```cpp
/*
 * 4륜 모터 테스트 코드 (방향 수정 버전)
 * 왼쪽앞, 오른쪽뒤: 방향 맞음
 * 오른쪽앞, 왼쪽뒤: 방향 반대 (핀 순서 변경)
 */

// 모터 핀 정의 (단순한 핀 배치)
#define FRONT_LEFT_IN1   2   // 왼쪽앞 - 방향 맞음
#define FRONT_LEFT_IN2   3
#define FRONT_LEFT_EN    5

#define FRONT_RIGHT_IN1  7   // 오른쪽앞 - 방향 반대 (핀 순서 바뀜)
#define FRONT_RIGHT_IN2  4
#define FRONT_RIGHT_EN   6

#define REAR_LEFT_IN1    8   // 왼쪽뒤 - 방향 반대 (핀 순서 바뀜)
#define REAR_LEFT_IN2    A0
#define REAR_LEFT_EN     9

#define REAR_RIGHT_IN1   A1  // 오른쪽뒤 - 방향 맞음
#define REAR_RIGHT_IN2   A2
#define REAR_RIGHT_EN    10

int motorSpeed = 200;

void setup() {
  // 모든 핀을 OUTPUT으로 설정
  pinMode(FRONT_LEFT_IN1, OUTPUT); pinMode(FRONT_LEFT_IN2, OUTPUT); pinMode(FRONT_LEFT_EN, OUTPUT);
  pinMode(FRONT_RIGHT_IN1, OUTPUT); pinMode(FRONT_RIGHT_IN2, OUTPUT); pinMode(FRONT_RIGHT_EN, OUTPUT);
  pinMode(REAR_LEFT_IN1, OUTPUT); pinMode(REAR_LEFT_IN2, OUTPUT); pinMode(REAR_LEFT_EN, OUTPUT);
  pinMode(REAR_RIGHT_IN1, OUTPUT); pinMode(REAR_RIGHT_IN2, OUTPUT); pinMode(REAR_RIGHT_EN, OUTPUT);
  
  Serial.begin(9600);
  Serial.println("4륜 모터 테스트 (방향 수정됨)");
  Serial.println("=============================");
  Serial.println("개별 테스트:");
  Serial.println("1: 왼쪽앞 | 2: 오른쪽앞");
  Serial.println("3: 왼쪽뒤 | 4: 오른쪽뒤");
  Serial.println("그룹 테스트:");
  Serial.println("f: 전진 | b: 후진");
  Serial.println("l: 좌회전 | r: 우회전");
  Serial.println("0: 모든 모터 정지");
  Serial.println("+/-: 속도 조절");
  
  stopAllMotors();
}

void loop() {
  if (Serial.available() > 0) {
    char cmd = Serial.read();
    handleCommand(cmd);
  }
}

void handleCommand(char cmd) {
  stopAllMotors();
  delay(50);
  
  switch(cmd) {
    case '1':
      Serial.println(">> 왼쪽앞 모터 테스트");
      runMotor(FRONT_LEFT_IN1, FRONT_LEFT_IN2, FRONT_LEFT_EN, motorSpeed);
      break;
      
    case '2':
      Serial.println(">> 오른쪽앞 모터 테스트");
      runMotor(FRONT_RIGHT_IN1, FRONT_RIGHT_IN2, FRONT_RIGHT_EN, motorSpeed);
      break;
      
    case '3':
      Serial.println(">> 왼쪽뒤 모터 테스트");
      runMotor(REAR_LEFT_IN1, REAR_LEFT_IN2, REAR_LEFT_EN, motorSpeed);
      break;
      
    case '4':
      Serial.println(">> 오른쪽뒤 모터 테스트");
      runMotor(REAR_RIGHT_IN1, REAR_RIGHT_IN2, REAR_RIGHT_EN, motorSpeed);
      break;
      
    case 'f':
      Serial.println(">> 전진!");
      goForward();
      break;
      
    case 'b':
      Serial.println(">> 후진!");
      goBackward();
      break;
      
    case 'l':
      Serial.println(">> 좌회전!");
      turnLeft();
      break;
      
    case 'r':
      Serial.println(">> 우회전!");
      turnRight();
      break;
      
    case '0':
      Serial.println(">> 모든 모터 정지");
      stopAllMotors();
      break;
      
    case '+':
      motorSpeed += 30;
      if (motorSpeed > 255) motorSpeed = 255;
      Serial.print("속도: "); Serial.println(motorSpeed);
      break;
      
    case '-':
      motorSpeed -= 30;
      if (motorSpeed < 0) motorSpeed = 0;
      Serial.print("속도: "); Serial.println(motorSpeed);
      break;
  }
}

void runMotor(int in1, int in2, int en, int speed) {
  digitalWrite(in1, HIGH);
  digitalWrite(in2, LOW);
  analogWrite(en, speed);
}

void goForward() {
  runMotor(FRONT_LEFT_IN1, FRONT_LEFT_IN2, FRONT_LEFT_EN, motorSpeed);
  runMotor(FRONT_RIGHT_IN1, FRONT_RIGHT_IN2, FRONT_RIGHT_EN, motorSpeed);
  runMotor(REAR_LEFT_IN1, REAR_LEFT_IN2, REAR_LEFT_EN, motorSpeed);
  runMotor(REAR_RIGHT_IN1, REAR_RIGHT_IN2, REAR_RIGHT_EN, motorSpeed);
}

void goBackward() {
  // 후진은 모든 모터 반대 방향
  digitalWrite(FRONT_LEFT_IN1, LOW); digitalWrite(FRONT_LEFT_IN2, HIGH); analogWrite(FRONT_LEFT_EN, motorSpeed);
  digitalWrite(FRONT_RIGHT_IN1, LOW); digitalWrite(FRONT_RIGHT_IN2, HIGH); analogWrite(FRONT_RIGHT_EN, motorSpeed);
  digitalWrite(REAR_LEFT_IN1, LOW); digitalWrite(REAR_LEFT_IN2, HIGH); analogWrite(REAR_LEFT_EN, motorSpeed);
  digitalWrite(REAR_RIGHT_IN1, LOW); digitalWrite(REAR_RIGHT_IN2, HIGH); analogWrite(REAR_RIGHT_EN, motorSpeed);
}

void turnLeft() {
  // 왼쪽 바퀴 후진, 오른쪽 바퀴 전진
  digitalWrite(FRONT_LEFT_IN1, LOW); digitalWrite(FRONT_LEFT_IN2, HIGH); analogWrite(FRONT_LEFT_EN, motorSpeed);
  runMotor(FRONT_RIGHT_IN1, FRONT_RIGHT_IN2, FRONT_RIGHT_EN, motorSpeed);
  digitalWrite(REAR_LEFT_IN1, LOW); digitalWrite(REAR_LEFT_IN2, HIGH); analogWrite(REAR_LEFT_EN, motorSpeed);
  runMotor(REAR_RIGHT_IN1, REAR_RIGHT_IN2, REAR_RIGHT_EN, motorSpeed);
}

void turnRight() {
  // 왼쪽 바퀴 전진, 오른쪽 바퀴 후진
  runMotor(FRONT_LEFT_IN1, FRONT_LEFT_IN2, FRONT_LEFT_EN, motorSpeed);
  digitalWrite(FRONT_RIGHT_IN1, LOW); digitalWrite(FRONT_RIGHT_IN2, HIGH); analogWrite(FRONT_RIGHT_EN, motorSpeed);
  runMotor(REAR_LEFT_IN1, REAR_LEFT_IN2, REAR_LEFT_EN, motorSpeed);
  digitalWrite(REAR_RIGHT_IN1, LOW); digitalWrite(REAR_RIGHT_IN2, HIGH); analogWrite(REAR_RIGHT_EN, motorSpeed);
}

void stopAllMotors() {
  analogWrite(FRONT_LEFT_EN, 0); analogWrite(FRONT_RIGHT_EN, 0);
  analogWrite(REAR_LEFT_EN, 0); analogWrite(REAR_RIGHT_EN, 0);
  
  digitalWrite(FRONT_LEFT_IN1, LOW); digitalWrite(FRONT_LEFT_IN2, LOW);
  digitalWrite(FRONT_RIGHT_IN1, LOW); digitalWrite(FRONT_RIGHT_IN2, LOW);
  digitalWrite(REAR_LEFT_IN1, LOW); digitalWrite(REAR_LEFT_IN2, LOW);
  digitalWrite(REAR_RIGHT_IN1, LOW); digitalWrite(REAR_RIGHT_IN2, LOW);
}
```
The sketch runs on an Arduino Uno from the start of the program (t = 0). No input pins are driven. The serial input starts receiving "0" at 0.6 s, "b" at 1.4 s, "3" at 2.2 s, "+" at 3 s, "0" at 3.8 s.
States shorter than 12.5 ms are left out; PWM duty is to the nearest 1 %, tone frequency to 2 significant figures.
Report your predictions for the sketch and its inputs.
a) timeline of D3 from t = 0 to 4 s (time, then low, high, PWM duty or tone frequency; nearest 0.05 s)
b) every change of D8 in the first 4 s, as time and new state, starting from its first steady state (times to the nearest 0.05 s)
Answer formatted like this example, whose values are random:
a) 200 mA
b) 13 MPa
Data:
a) 0 s low; 1.45 s high; 2.2 s low
b) 0 s low; 2.25 s high; 3 s low
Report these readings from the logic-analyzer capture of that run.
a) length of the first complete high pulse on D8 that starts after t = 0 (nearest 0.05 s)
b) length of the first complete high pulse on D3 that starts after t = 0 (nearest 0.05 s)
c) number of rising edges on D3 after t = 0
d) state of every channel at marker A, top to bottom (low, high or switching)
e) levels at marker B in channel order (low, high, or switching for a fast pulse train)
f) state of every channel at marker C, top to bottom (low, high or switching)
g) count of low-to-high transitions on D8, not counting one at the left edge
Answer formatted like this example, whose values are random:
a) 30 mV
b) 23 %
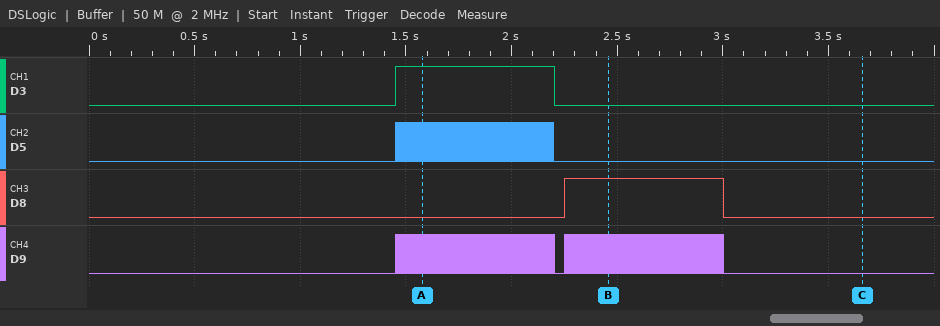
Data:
a) 0.75 s
b) 0.75 s
c) 1
d) D3 high, D5 switching, D8 low, D9 switching
e) D3 low, D5 low, D8 high, D9 switching
f) D3 low, D5 low, D8 low, D9 low
g) 1
